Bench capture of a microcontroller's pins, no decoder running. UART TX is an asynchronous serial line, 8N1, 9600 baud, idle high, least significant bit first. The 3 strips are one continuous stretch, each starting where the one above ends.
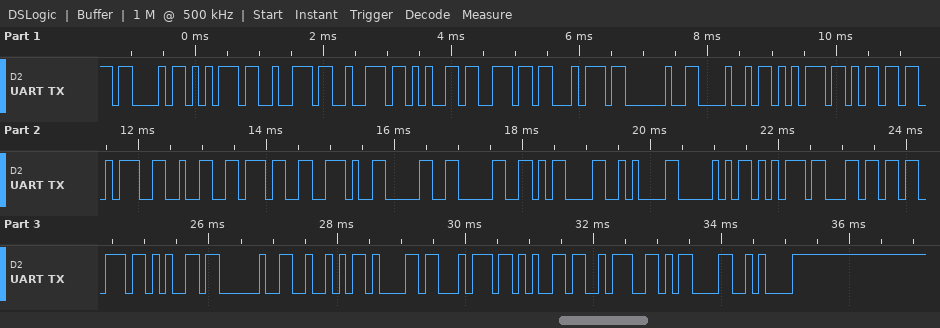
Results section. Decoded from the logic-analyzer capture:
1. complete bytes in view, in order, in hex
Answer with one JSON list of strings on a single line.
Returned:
["0x43 0x75 0x72 0x72 0x65 0x6E 0x74 0x20 0x48 0x75 0x6D 0x3A 0x32 0x37 0x2E 0x30 0x30 0x0D 0x0A 0x50 0x75 0x6C 0x73 0x65 0x20 0x52 0x61 0x74 0x65 0x3A 0x0D 0x0A"]
